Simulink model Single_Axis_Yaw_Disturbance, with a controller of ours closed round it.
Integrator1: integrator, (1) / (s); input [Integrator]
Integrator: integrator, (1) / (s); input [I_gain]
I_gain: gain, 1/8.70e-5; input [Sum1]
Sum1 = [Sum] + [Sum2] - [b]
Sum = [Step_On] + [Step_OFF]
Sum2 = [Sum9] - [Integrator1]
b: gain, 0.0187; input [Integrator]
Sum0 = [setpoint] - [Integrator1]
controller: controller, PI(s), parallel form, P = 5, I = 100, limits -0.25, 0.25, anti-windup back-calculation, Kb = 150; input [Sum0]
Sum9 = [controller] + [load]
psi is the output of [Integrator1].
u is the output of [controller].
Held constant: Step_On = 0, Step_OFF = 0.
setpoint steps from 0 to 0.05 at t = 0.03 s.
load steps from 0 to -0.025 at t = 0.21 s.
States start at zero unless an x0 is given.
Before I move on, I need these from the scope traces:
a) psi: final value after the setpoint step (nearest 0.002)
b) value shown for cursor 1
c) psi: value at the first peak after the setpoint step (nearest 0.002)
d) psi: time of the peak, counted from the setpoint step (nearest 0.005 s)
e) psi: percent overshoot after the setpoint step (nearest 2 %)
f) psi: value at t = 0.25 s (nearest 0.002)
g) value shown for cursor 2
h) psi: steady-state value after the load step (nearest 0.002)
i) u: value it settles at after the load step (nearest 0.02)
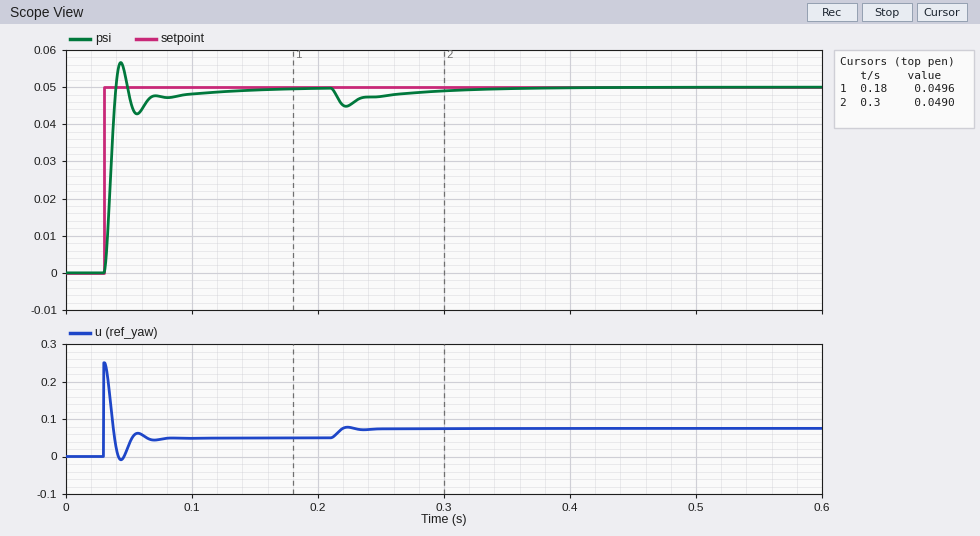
0.050
0.0496
0.056
0.015 s
14 %
0.048
0.0490
0.050
0.08
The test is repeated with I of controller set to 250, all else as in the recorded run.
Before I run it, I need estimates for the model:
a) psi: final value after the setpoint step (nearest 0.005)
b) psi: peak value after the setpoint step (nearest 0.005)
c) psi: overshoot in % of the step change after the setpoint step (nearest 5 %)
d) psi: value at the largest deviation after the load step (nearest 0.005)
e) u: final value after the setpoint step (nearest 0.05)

0.050
0.065
25 %
0.045
0.05
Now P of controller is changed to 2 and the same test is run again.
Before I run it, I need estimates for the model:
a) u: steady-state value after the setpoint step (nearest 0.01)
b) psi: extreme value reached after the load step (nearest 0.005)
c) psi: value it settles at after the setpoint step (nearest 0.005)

0.05
0.040
0.050
